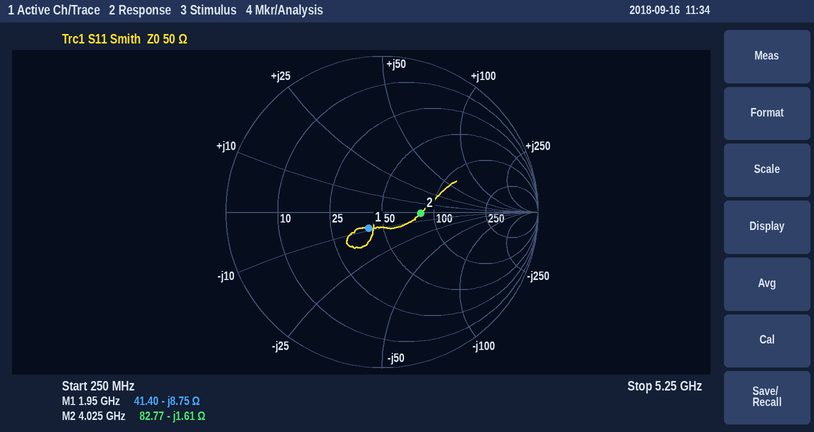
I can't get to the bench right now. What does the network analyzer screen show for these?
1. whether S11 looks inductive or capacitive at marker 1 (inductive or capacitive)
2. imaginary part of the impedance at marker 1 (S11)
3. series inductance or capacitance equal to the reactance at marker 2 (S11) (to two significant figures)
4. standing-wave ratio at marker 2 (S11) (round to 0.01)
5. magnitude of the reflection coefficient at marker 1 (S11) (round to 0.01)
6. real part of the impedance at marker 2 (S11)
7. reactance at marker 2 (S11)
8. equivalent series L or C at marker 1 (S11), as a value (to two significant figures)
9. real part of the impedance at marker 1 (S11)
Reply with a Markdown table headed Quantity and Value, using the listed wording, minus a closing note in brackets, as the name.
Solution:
| Quantity | Value |
|---|---|
| whether S11 looks inductive or capacitive at marker 1 | capacitive |
| imaginary part of the impedance at marker 1 | -8.75 Ω |
| series inductance or capacitance equal to the reactance at marker 2 (S11) | 25 pF |
| standing-wave ratio at marker 2 (S11) | 1.66 |
| magnitude of the reflection coefficient at marker 1 (S11) | 0.13 |
| real part of the impedance at marker 2 | 82.77 Ω |
| reactance at marker 2 | -1.61 Ω |
| equivalent series L or C at marker 1 (S11), as a value | 9.3 pF |
| real part of the impedance at marker 1 | 41.40 Ω |
